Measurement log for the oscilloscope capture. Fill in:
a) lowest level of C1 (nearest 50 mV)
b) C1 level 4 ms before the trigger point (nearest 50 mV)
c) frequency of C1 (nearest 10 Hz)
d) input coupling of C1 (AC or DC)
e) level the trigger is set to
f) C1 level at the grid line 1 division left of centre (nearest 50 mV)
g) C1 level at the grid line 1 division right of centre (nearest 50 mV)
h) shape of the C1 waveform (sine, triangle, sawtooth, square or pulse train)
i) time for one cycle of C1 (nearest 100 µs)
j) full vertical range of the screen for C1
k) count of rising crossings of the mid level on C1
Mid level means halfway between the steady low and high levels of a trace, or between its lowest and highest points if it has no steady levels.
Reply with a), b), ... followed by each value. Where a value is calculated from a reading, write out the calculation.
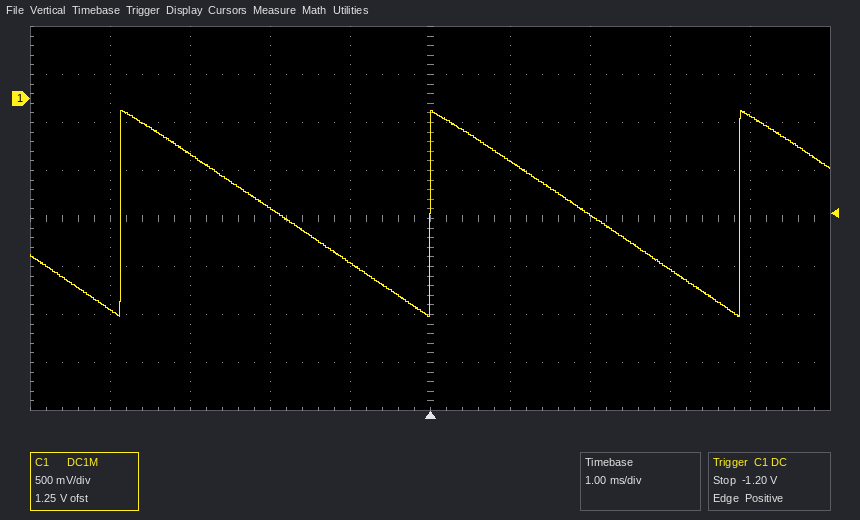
a) -2.25 V
b) -2.20 V
c) 1 / 3.9 ms ≈ 256 Hz, so 260 Hz to the nearest 10 Hz
d) DC
e) -1.20 V
f) -1.70 V
g) -650 mV
h) sawtooth
i) 3.9 ms
j) 4 V
k) 3
